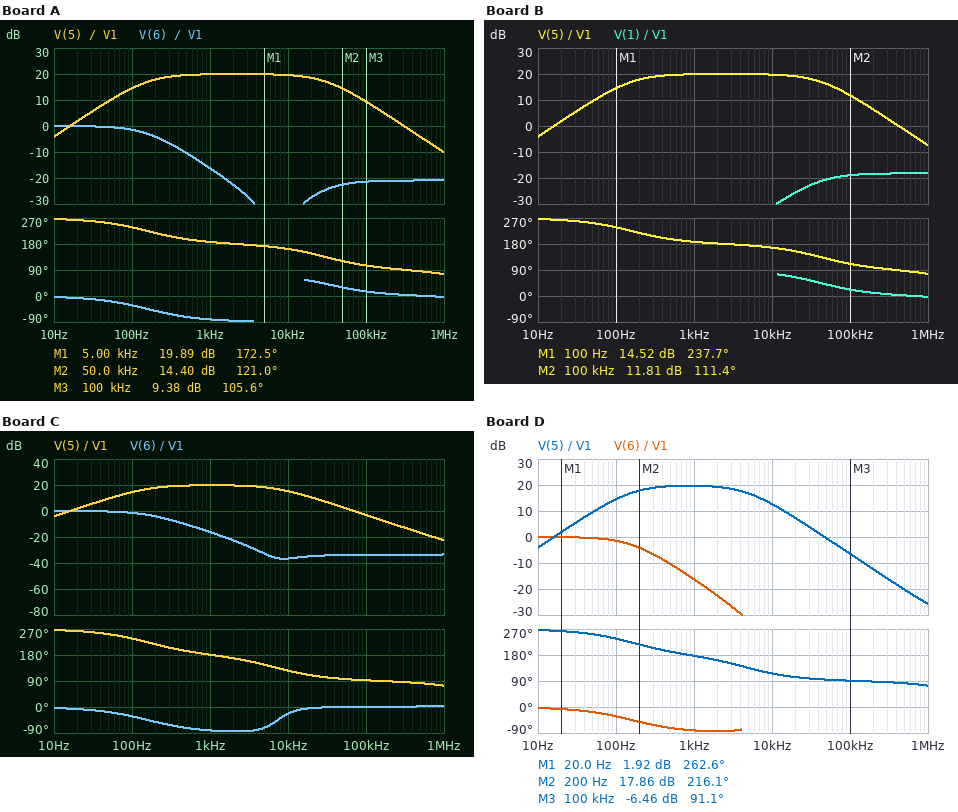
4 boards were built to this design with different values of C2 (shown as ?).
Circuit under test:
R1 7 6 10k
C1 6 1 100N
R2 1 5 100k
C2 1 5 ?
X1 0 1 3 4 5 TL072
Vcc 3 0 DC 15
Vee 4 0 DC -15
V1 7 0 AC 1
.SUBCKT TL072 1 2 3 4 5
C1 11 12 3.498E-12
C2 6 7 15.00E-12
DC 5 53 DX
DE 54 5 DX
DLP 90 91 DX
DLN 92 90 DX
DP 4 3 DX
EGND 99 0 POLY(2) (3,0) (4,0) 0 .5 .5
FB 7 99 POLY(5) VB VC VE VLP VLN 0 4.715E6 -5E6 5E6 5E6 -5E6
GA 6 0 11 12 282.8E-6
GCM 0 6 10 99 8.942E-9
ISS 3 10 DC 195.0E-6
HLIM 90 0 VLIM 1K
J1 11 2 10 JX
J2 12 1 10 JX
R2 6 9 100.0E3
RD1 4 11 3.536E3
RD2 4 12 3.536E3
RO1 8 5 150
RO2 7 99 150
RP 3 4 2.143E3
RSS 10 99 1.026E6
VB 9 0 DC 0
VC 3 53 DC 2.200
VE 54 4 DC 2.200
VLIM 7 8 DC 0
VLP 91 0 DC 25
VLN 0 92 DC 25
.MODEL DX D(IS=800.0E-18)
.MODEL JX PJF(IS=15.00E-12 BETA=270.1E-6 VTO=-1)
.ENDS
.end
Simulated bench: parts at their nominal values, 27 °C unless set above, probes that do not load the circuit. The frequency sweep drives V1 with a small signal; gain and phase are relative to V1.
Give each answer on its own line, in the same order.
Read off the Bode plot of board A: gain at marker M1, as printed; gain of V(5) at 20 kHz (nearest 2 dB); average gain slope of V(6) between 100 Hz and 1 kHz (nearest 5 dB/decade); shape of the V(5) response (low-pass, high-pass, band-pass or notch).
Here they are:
19.89 dB
18 dB
-15 dB/decade
band-pass
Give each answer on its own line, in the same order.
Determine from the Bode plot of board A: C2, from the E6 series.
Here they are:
47 pF
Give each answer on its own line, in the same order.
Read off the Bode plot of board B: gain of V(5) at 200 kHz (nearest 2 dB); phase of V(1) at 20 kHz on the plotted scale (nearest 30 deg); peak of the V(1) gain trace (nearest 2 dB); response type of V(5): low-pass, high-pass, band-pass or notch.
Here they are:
6 dB
60 deg
-18 dB
band-pass
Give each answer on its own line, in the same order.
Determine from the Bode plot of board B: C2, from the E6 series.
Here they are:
33 pF
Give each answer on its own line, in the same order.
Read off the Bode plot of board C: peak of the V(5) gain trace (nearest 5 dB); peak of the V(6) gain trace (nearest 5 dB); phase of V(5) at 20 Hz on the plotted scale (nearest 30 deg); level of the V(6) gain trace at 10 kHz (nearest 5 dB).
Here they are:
20 dB
0 dB
270 deg
-35 dB
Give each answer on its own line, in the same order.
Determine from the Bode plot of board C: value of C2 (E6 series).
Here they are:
220 pF
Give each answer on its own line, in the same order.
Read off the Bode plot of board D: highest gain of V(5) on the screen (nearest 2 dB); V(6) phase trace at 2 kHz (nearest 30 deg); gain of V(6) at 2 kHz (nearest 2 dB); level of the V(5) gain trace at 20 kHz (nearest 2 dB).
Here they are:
20 dB
-90 deg
-22 dB
8 dB
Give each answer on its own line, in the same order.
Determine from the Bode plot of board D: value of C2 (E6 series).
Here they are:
330 pF
